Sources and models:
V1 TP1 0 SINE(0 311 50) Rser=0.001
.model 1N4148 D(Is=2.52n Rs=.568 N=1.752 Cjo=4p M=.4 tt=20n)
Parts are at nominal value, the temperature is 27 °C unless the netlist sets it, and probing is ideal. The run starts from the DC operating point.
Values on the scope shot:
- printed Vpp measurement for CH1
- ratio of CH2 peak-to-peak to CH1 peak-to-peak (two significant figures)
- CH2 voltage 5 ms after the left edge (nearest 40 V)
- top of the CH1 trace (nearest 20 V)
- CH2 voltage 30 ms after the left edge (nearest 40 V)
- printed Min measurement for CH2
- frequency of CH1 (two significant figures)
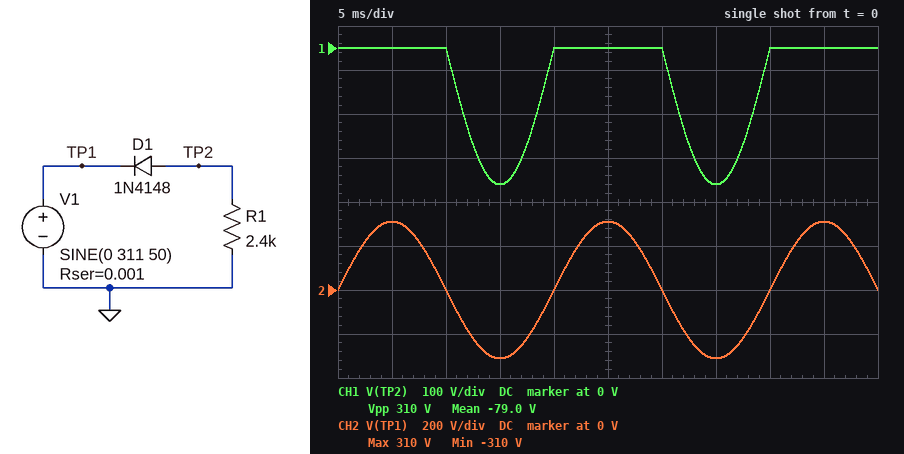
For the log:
310 V
2.0
320 V
0 V
0 V
-310 V
50 Hz
